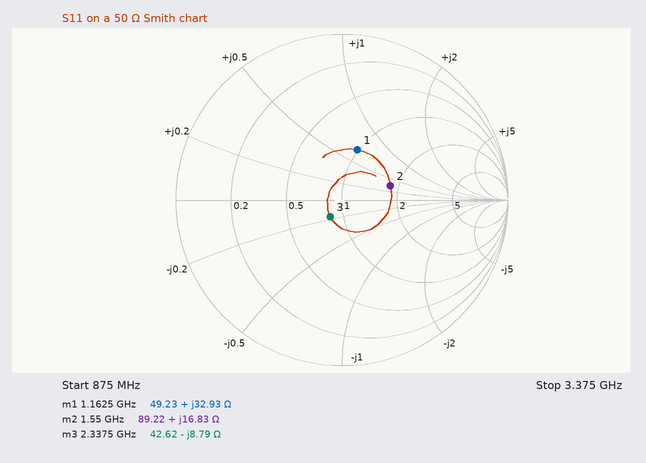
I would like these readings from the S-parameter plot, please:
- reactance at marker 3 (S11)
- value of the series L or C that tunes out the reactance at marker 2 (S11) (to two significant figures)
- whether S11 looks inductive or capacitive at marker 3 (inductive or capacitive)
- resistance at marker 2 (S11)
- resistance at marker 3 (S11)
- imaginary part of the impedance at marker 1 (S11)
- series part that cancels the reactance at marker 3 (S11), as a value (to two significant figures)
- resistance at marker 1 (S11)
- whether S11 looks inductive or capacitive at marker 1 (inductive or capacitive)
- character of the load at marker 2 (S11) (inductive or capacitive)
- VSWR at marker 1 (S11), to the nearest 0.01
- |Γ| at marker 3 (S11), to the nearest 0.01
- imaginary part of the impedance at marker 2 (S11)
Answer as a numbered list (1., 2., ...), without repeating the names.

1. -8.79 Ω
2. 6.1 pF
3. capacitive
4. 89.22 Ω
5. 42.62 Ω
6. +32.93 Ω
7. 600 pH
8. 49.23 Ω
9. inductive
10. inductive
11. 1.92
12. 0.12
13. +16.83 Ω
